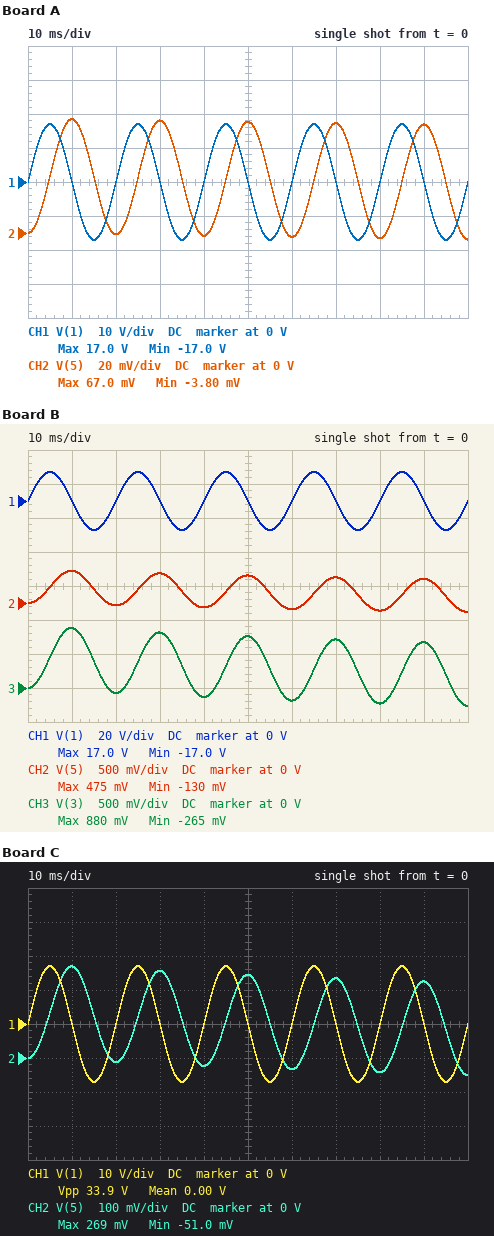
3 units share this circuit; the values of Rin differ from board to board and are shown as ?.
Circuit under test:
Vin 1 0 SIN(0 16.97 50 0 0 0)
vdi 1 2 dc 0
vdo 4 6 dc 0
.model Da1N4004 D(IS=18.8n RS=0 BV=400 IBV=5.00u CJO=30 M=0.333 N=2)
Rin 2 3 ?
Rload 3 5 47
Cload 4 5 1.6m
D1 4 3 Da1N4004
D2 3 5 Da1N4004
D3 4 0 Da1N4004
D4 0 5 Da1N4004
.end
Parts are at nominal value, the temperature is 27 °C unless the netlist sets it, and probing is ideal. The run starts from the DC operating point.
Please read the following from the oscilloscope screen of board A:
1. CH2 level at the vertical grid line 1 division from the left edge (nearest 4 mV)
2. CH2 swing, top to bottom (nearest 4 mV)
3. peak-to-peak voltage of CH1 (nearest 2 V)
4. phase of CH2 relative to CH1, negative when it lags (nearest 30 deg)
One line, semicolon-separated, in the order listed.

68 mV; 72 mV; 34 V; -90 deg
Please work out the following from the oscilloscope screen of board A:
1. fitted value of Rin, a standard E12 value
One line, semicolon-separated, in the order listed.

0.027 Ω
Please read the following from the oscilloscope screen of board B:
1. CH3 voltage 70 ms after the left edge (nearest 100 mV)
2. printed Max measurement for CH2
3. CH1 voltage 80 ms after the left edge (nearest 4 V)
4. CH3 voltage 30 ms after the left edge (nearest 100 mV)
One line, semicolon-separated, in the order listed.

700 mV; 475 mV; 0 V; 800 mV
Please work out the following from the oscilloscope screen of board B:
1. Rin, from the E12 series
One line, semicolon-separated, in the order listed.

3.9 mΩ
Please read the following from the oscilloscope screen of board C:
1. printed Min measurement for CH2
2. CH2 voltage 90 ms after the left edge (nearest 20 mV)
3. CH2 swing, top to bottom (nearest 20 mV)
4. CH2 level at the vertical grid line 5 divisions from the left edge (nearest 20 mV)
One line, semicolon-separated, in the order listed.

-51.0 mV; 220 mV; 320 mV; 240 mV
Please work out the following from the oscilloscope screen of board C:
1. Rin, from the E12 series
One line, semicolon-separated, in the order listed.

6.8 mΩ
